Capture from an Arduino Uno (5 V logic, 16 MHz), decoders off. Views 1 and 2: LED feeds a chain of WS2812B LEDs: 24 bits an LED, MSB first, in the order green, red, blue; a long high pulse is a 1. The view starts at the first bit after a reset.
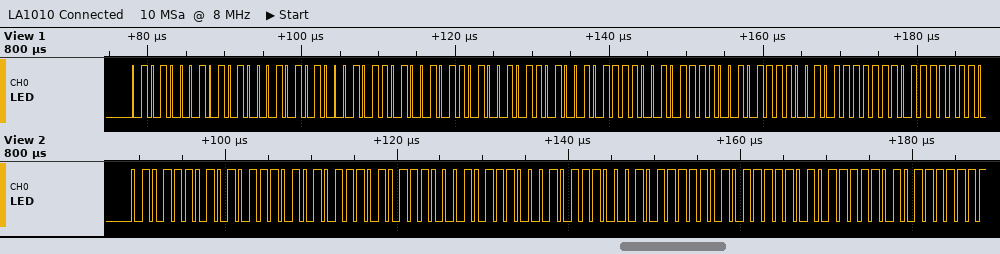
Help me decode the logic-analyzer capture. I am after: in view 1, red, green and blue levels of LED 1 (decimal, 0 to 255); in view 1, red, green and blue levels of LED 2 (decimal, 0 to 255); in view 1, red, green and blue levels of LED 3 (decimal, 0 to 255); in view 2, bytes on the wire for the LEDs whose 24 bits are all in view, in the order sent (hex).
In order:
81, 81, 81
105, 105, 105
121, 121, 121
5D 5D 5D 71 71 71 7D 7D 7D
